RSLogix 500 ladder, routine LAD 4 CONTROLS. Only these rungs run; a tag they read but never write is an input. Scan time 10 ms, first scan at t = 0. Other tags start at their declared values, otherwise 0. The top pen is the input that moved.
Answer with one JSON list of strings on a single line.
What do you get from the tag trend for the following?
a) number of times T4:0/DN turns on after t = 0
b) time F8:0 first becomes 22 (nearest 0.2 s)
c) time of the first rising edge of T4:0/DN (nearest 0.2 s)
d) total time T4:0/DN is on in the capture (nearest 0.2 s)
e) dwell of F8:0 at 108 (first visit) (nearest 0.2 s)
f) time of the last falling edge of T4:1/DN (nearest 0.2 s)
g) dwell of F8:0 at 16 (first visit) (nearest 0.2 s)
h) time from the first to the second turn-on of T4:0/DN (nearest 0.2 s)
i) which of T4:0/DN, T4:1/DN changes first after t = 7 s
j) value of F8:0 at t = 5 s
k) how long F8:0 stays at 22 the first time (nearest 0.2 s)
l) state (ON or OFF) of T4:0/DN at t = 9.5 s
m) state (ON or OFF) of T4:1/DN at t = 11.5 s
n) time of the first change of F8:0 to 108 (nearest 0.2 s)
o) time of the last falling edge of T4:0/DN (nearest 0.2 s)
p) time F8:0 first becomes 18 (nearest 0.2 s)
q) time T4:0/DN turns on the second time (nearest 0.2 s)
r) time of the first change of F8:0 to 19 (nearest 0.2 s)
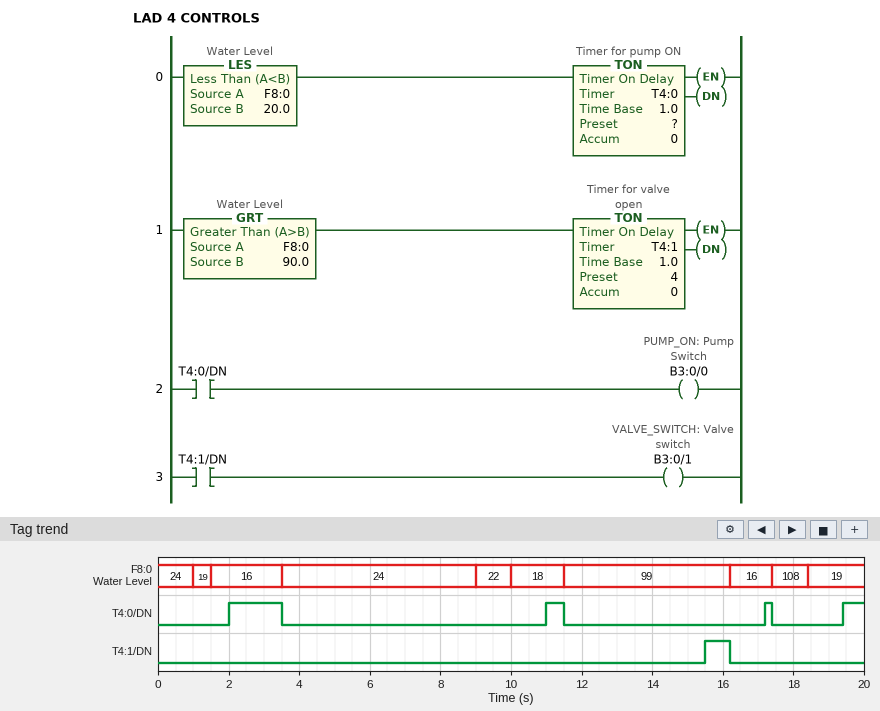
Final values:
["4", "9.0 s", "2.0 s", "2.8 s", "1.0 s", "16.2 s", "2.0 s", "9.0 s", "T4:0/DN", "24", "1.0 s", "OFF", "OFF", "17.4 s", "17.4 s", "10.0 s", "11.0 s", "1.0 s"]
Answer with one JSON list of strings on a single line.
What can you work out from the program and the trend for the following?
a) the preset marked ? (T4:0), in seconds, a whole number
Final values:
["1 s"]
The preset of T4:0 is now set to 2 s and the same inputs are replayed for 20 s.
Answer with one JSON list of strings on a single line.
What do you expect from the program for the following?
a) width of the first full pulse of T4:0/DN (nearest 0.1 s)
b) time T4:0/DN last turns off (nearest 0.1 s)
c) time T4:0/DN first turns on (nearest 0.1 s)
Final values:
["0.5 s", "3.5 s", "3.0 s"]
